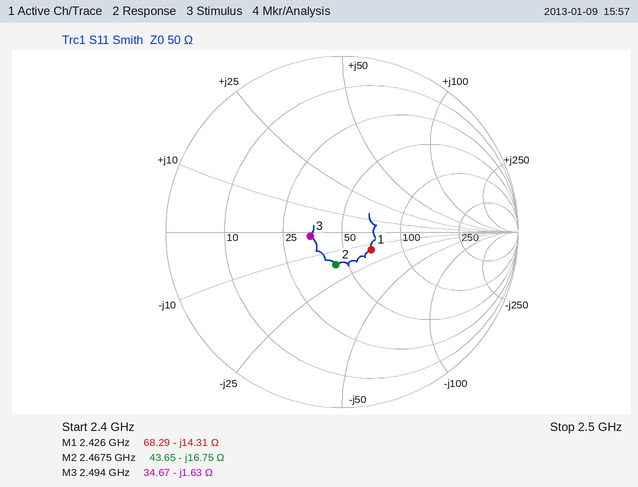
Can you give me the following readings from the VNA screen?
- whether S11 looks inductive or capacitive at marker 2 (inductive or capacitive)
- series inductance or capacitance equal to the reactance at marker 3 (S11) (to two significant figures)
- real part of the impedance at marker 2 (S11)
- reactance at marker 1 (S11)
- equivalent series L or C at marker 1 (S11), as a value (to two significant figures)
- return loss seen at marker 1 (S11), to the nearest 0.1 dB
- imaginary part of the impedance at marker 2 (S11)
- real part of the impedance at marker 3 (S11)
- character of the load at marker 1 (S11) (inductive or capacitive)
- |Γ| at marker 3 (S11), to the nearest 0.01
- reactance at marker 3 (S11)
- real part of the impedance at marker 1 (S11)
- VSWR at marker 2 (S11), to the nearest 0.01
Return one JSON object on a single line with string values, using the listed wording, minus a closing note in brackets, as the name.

{"whether S11 looks inductive or capacitive at marker 2": "capacitive", "series inductance or capacitance equal to the reactance at marker 3 (S11)": "39 pF", "real part of the impedance at marker 2": "43.65 Ω", "reactance at marker 1": "-14.31 Ω", "equivalent series L or C at marker 1 (S11), as a value": "4.6 pF", "return loss seen at marker 1 (S11), to the nearest 0.1 dB": "14.2 dB", "imaginary part of the impedance at marker 2": "-16.75 Ω", "real part of the impedance at marker 3": "34.67 Ω", "character of the load at marker 1 (S11)": "capacitive", "|Γ| at marker 3 (S11), to the nearest 0.01": "0.18", "reactance at marker 3": "-1.63 Ω", "real part of the impedance at marker 1": "68.29 Ω", "VSWR at marker 2 (S11), to the nearest 0.01": "1.46"}
